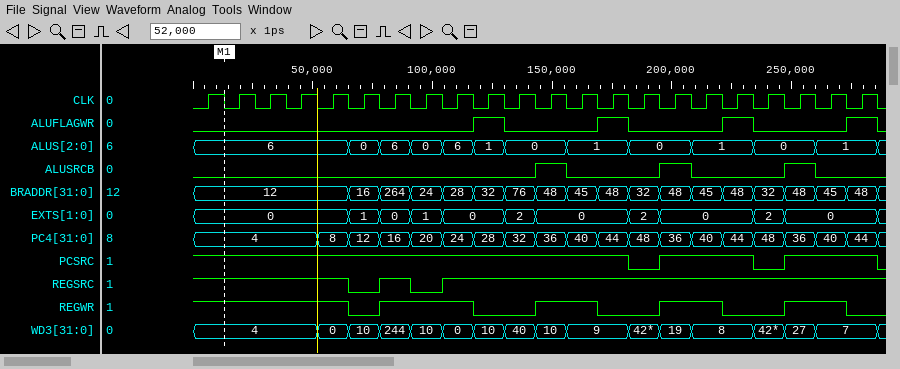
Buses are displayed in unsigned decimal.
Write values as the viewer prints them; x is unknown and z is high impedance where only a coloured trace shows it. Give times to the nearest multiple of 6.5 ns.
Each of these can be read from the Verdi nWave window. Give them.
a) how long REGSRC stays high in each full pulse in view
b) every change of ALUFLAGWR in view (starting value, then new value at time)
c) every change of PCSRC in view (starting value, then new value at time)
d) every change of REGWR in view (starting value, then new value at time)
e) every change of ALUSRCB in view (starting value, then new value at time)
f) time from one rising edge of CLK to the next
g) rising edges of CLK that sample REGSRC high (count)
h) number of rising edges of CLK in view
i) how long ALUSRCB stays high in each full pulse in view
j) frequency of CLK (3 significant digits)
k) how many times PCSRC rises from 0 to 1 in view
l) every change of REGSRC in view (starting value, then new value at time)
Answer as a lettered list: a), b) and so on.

a) 13 ns
b) 0, 1 at 117 ns, 0 at 130 ns, 1 at 169 ns, 0 at 182 ns, 1 at 221 ns, 0 at 234 ns, 1 at 273 ns, 0 at 286 ns
c) 1, 0 at 182 ns, 1 at 195 ns, 0 at 234 ns, 1 at 247 ns, 0 at 286 ns
d) 1, 0 at 65 ns, 1 at 78 ns, 0 at 117 ns, 1 at 143 ns, 0 at 169 ns, 1 at 195 ns, 0 at 221 ns, 1 at 247 ns, 0 at 273 ns
e) 0, 1 at 143 ns, 0 at 156 ns, 1 at 195 ns, 0 at 208 ns, 1 at 247 ns, 0 at 260 ns
f) 13 ns
g) 20
h) 22
i) 13 ns, 13 ns, 13 ns
j) 76.9 MHz
k) 2
l) 1, 0 at 65 ns, 1 at 78 ns, 0 at 91 ns, 1 at 104 ns
